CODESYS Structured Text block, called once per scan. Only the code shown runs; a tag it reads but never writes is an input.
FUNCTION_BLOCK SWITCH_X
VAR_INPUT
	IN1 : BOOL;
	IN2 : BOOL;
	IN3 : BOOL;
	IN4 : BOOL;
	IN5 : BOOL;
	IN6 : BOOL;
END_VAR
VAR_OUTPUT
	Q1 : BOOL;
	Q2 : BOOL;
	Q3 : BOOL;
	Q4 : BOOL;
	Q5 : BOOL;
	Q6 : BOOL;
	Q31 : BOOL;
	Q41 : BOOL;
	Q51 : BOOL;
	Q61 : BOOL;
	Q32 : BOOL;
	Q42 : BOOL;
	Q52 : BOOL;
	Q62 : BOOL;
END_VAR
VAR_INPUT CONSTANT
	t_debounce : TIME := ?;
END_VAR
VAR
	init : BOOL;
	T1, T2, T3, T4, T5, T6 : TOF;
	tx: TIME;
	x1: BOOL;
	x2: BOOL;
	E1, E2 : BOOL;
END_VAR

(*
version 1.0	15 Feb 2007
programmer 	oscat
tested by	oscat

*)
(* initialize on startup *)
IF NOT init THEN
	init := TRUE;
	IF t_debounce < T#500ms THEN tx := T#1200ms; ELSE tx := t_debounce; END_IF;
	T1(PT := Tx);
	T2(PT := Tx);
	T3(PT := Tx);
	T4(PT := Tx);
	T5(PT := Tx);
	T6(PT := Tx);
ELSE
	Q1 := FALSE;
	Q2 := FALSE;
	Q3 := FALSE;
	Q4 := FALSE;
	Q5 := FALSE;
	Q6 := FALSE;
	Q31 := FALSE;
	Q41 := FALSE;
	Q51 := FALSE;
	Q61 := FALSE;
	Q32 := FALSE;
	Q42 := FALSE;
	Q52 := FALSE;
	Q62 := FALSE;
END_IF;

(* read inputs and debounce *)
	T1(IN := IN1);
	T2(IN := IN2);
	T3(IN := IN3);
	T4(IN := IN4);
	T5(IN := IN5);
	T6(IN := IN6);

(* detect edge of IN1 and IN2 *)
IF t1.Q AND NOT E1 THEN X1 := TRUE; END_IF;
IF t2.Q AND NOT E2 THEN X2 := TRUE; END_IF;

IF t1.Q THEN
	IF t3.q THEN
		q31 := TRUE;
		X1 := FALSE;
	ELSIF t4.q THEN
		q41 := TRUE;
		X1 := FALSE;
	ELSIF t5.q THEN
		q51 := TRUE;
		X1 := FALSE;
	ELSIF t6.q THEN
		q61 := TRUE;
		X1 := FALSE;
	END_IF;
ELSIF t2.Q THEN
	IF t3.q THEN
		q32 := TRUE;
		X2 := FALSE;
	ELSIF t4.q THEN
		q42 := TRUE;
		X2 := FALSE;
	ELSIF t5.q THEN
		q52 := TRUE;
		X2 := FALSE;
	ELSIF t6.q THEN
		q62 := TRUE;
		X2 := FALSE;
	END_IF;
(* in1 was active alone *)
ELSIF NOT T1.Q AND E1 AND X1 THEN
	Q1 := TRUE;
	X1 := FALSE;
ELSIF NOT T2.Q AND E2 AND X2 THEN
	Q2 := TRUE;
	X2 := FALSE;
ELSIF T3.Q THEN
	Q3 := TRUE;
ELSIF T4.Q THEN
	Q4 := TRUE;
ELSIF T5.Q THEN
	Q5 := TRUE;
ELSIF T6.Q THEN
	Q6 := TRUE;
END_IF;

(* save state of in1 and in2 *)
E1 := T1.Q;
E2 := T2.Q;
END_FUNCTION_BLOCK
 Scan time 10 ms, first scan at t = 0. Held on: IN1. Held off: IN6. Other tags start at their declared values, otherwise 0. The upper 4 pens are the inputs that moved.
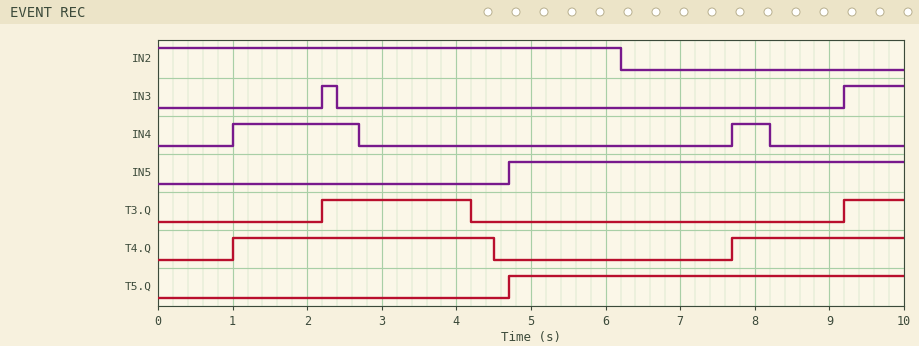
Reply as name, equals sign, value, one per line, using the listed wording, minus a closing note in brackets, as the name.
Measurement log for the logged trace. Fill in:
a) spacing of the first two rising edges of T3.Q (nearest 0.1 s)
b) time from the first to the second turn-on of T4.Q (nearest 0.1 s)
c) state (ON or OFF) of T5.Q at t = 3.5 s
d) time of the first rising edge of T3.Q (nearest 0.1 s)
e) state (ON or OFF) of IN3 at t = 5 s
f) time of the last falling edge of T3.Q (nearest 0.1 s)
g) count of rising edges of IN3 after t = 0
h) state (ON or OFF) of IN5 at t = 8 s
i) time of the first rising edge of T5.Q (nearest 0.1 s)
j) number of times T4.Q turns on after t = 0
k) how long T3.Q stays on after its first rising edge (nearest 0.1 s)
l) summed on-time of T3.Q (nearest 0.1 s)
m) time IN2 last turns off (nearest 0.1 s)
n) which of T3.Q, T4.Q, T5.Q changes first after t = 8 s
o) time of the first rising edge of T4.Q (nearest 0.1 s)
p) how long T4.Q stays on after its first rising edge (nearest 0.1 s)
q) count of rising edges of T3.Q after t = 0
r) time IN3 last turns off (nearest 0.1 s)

spacing of the first two rising edges of T3.Q = 7.0 s
time from the first to the second turn-on of T4.Q = 6.7 s
state (ON or OFF) of T5.Q at t = 3.5 s = OFF
time of the first rising edge of T3.Q = 2.2 s
state (ON or OFF) of IN3 at t = 5 s = OFF
time of the last falling edge of T3.Q = 4.2 s
count of rising edges of IN3 after t = 0 = 2
state (ON or OFF) of IN5 at t = 8 s = ON
time of the first rising edge of T5.Q = 4.7 s
number of times T4.Q turns on after t = 0 = 2
how long T3.Q stays on after its first rising edge = 2.0 s
summed on-time of T3.Q = 2.8 s
time IN2 last turns off = 6.2 s
which of T3.Q, T4.Q, T5.Q changes first after t = 8 s = T3.Q
time of the first rising edge of T4.Q = 1.0 s
how long T4.Q stays on after its first rising edge = 3.5 s
count of rising edges of T3.Q after t = 0 = 2
time IN3 last turns off = 2.4 s
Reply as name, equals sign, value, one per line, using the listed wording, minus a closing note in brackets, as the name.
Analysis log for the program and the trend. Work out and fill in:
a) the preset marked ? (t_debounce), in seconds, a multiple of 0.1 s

the preset marked ? (t_debounce), in seconds, a multiple of 0.1 s = 1.8 s
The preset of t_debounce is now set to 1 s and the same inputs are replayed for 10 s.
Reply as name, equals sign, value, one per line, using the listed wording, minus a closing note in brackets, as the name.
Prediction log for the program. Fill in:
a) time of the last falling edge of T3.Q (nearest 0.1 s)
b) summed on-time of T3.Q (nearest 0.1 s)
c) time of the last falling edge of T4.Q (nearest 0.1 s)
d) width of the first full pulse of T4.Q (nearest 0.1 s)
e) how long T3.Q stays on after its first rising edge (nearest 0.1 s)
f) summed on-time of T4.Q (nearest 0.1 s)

time of the last falling edge of T3.Q = 3.4 s
summed on-time of T3.Q = 2.0 s
time of the last falling edge of T4.Q = 9.2 s
width of the first full pulse of T4.Q = 2.7 s
how long T3.Q stays on after its first rising edge = 1.2 s
summed on-time of T4.Q = 4.2 s
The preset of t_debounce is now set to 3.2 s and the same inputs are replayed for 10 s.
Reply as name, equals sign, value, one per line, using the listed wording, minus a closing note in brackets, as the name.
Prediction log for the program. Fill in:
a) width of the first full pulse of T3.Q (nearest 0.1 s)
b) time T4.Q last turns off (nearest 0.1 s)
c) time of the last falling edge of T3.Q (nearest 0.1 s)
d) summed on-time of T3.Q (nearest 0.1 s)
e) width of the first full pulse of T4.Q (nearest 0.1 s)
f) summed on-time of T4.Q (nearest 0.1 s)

width of the first full pulse of T3.Q = 3.4 s
time T4.Q last turns off = 5.9 s
time of the last falling edge of T3.Q = 5.6 s
summed on-time of T3.Q = 4.2 s
width of the first full pulse of T4.Q = 4.9 s
summed on-time of T4.Q = 7.2 s
